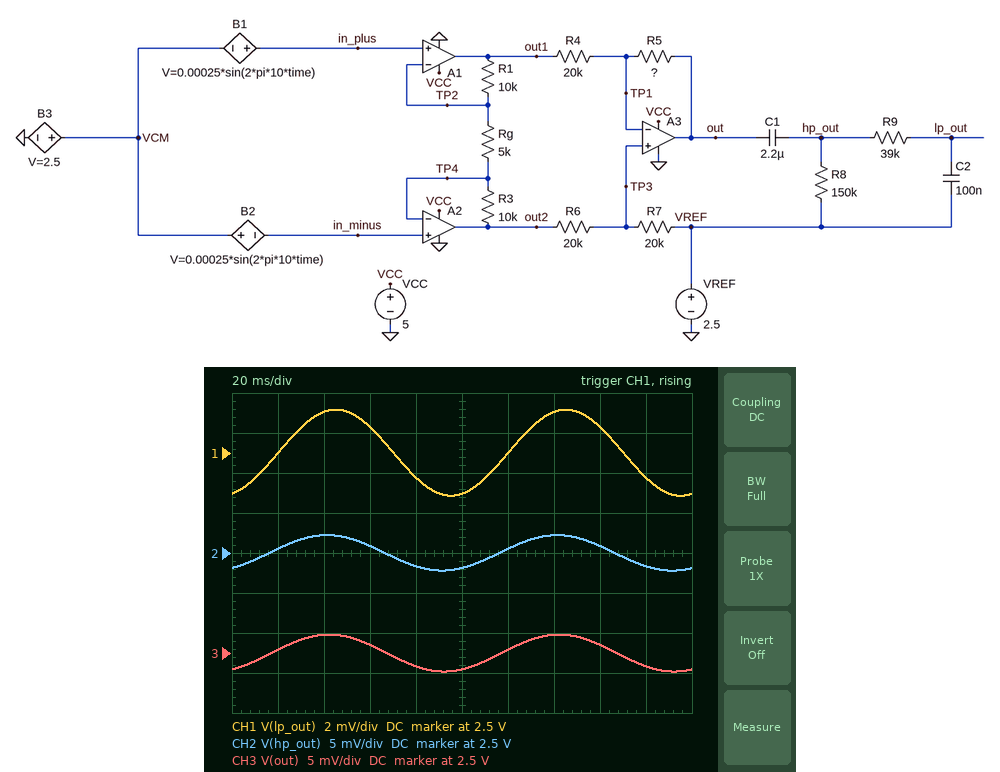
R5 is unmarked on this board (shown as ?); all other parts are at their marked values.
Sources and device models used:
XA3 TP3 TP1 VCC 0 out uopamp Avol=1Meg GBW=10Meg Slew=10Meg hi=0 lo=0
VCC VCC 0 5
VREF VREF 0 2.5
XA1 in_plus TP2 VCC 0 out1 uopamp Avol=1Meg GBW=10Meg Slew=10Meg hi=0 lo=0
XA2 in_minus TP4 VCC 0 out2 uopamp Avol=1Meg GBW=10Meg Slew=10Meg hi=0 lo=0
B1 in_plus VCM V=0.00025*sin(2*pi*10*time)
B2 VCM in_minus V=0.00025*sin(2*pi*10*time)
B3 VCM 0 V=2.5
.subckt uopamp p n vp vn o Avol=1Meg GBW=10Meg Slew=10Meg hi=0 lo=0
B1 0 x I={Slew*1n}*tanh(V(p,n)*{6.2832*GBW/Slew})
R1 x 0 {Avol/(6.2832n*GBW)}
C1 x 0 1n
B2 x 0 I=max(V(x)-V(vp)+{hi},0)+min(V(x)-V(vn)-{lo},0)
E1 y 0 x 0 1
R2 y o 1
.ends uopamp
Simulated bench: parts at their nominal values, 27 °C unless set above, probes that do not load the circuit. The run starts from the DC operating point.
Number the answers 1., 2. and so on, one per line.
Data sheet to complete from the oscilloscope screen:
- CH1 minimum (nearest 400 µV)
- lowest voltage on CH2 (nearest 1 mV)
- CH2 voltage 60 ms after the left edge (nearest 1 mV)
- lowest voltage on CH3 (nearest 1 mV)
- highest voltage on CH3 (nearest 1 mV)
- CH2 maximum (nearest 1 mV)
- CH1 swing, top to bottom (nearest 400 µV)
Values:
1. 2.4980 V
2. 2.498 V
3. 2.501 V
4. 2.498 V
5. 2.502 V
6. 2.502 V
7. 4.4 mV
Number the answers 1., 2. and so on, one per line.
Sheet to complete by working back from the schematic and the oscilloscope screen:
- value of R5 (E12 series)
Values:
1. 18 kΩ
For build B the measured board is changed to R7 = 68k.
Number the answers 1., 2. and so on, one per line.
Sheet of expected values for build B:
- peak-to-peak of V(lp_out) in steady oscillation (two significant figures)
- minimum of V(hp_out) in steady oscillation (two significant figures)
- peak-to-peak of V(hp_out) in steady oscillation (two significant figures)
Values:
1. 5.5 mV
2. 2.5 V
3. 5.7 mV
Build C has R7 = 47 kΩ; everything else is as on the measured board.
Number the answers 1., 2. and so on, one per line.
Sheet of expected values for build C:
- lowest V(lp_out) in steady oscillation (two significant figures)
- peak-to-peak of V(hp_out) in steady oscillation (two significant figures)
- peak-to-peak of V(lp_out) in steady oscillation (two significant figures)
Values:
1. 2.5 V
2. 5.4 mV
3. 5.2 mV
